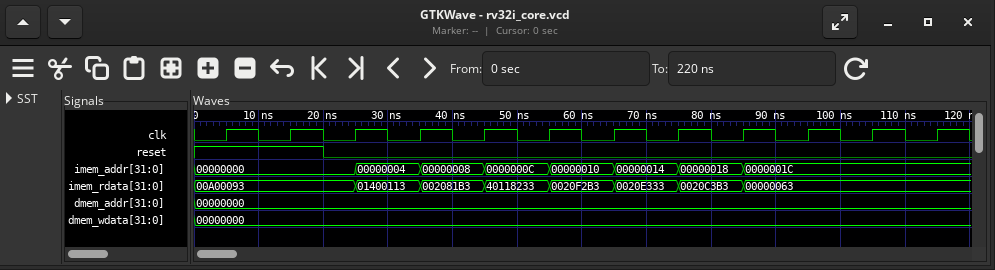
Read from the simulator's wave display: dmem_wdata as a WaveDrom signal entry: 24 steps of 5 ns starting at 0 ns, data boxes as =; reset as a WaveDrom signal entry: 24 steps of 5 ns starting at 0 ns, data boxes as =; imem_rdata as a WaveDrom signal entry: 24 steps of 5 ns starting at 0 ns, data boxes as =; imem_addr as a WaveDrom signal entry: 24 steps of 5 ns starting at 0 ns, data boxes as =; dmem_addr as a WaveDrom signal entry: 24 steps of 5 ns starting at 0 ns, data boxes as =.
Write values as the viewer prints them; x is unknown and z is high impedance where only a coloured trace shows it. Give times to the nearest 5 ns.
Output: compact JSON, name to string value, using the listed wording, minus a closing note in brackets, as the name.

{"dmem_wdata as a WaveDrom signal entry: 24 steps of 5 ns starting at 0 ns, data boxes as =": "{name: 'dmem_wdata', wave: '=.......................', data: '00000000'}", "reset as a WaveDrom signal entry: 24 steps of 5 ns starting at 0 ns, data boxes as =": "{name: 'reset', wave: '1...0...................'}", "imem_rdata as a WaveDrom signal entry: 24 steps of 5 ns starting at 0 ns, data boxes as =": "{name: 'imem_rdata', wave: '=....=.=.=.=.=.=.=......', data: '00A00093 01400113 002081B3 40118233 0020F2B3 0020E333 0020C3B3 00000063'}", "imem_addr as a WaveDrom signal entry: 24 steps of 5 ns starting at 0 ns, data boxes as =": "{name: 'imem_addr', wave: '=....=.=.=.=.=.=.=......', data: '00000000 00000004 00000008 0000000C 00000010 00000014 00000018 0000001C'}", "dmem_addr as a WaveDrom signal entry: 24 steps of 5 ns starting at 0 ns, data boxes as =": "{name: 'dmem_addr', wave: '=.......................', data: '00000000'}"}
